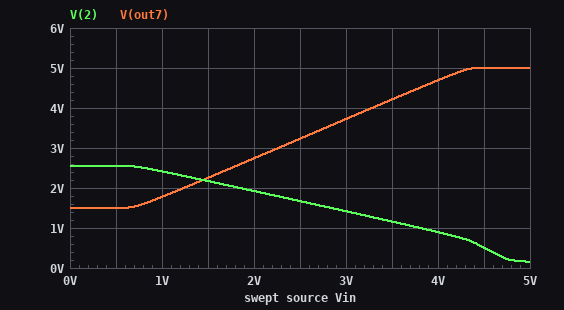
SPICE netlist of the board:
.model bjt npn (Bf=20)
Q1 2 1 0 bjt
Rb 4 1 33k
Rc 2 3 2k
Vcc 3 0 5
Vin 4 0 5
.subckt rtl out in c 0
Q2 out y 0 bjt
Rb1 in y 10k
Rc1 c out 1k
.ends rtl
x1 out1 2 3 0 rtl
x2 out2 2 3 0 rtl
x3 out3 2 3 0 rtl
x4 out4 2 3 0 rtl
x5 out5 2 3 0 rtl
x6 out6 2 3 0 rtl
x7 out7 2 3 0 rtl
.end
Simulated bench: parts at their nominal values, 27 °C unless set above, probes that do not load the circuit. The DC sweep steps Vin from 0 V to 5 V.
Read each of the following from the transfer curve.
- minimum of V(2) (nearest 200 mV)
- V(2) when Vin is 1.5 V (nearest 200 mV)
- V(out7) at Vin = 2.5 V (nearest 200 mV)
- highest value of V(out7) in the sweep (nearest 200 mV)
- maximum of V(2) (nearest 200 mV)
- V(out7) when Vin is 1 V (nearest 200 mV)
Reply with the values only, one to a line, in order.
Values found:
200 mV
2.2 V
3.2 V
5.0 V
2.6 V
1.8 V
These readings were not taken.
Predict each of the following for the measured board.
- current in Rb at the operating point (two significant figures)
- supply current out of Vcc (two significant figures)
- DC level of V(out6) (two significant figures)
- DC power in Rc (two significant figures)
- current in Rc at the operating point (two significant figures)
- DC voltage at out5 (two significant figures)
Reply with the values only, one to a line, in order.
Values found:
130 µA
2.4 mA
5.0 V
12 mW
2.4 mA
5.0 V
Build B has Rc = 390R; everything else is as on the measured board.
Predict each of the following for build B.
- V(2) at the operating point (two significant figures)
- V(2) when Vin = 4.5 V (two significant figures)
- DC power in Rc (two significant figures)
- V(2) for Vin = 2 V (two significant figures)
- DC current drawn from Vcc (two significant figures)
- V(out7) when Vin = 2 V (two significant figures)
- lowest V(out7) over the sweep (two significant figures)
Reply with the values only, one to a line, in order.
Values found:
3.3 V
3.4 V
7.2 mW
3.9 V
38 mA
120 mV
110 mV
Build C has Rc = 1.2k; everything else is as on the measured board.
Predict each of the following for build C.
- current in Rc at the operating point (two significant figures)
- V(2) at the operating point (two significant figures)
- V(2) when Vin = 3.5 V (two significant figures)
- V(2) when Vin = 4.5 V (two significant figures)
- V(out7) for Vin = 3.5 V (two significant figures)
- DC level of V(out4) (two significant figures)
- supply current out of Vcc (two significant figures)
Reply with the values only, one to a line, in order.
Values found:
3.0 mA
1.4 V
2.0 V
1.6 V
2.6 V
3.7 V
12 mA
